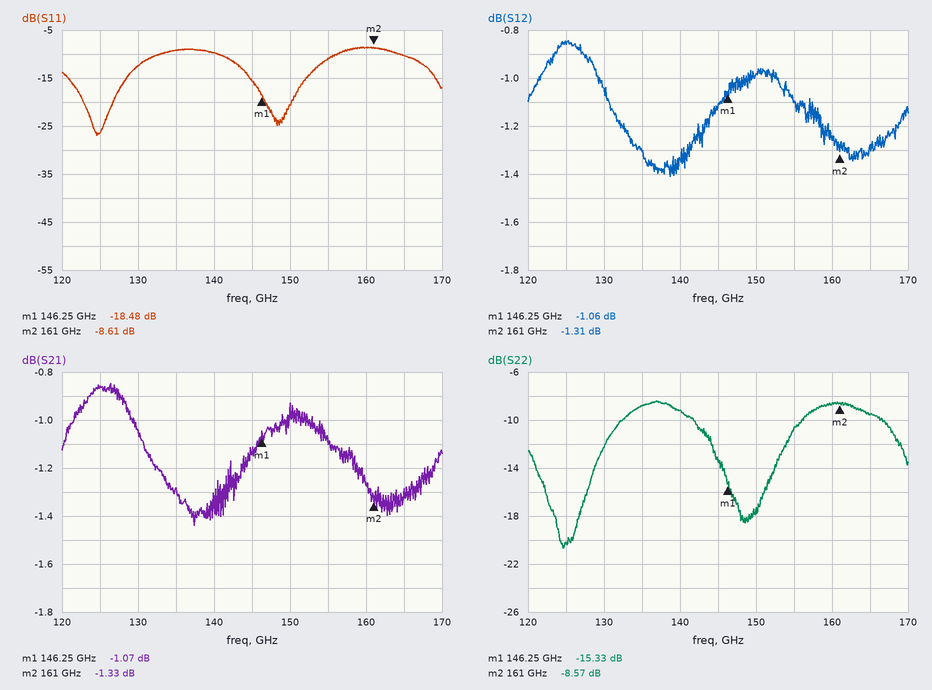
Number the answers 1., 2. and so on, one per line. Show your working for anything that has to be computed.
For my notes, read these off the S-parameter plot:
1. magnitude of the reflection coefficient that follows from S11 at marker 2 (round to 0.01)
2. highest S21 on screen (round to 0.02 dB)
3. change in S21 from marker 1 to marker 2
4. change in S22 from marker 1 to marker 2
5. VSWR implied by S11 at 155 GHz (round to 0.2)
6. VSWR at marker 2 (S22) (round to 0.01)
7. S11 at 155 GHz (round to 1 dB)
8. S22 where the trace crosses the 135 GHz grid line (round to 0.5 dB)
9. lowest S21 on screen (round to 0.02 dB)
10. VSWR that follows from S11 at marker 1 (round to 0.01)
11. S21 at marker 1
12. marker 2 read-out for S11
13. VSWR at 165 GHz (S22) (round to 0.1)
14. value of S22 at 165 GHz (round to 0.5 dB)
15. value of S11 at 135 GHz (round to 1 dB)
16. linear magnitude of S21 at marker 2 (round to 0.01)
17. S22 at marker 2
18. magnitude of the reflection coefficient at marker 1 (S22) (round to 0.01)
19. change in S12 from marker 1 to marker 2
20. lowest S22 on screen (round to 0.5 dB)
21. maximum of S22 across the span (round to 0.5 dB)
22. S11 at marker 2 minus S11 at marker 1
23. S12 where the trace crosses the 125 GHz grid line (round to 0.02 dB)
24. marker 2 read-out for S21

1. 10^(-8.61/20) ≈ 0.37
2. -0.84 dB
3. -1.33 − (-1.07) = -0.26 dB
4. -8.57 − (-15.33) = 6.76 dB
5. |Γ| = 10^(-11/20) = 0.2818; VSWR = (1 + 0.2818)/(1 − 0.2818) ≈ 1.8
6. (1 + 0.3728)/(1 − 0.3728) ≈ 2.19
7. -11 dB
8. -9.0 dB
9. -1.44 dB
10. (1 + 0.1191)/(1 − 0.1191) ≈ 1.27
11. -1.07 dB
12. -8.61 dB
13. |Γ| = 10^(-9.5/20) = 0.3350; VSWR = (1 + 0.3350)/(1 − 0.3350) ≈ 2.0
14. -9.5 dB
15. -9 dB
16. 10^(-1.33/20) ≈ 0.86
17. -8.57 dB
18. 10^(-15.33/20) ≈ 0.17
19. -1.31 − (-1.06) = -0.25 dB
20. -20.5 dB
21. -8.5 dB
22. -8.61 − (-18.48) = 9.87 dB
23. -0.86 dB
24. -1.33 dB
